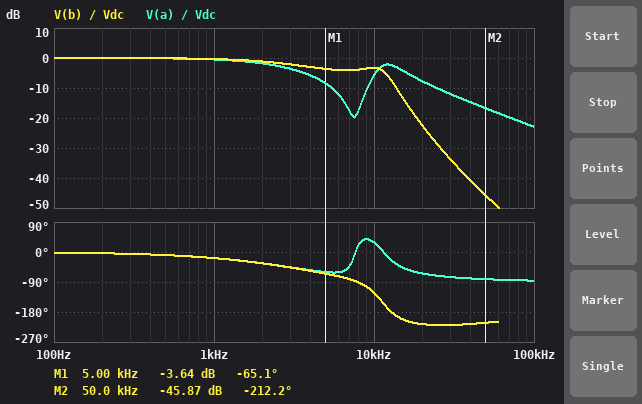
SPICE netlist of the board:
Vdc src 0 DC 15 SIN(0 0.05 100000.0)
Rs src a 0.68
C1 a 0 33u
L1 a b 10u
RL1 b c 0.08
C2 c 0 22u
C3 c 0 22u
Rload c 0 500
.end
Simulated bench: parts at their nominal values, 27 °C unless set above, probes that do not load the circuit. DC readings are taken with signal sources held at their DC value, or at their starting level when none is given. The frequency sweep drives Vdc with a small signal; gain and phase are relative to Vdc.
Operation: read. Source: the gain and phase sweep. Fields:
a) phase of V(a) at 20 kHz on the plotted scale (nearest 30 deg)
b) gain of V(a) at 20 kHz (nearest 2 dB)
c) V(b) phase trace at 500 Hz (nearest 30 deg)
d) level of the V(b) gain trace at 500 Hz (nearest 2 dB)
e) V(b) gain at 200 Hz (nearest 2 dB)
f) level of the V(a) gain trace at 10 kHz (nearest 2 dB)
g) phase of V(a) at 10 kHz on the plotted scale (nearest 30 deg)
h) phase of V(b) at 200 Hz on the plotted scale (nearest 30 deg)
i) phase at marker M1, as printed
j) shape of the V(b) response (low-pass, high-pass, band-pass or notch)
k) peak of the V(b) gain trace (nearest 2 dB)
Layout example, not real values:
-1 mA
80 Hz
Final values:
-60 deg
-8 dB
0 deg
0 dB
0 dB
-6 dB
30 deg
0 deg
-65.1 deg
low-pass
0 dB
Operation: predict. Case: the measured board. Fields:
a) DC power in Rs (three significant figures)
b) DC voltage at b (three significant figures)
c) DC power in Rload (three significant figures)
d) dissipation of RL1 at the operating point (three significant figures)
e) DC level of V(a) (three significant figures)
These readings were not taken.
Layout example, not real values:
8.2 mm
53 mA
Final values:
610 µW
15.0 V
449 mW
71.8 µW
15.0 V
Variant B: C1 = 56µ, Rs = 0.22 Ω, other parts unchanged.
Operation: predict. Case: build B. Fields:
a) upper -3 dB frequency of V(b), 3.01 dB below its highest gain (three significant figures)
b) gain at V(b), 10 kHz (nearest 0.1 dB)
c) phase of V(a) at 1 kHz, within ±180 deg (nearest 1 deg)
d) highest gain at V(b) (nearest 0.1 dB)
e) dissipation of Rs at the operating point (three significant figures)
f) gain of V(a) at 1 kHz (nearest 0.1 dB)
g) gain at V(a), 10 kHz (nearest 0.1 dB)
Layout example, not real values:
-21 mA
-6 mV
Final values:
9.86 kHz
0.7 dB
-8 deg
4.1 dB
198 µW
-0.1 dB
-1.8 dB
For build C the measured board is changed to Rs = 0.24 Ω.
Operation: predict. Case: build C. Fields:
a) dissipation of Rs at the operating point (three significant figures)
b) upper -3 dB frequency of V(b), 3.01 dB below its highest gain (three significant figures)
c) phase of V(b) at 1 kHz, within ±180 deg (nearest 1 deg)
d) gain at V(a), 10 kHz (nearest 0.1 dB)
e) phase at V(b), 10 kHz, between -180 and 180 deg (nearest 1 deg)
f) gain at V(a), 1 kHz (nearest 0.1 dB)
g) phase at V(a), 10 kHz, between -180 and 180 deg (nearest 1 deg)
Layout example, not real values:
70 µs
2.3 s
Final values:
216 µW
9.87 kHz
-7 deg
-2.2 dB
-136 deg
-0.1 dB
15 deg
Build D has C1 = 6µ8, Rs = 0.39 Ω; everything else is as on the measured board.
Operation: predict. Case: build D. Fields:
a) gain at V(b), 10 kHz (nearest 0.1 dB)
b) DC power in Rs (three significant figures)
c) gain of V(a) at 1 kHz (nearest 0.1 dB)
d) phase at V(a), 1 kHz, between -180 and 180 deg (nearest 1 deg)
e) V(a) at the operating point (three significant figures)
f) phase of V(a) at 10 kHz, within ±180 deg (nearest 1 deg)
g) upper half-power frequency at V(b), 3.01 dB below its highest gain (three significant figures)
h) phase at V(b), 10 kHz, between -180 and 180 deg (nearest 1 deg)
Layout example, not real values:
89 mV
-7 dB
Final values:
-2.8 dB
350 µW
-0.1 dB
-7 deg
15.0 V
40 deg
9.42 kHz
-111 deg
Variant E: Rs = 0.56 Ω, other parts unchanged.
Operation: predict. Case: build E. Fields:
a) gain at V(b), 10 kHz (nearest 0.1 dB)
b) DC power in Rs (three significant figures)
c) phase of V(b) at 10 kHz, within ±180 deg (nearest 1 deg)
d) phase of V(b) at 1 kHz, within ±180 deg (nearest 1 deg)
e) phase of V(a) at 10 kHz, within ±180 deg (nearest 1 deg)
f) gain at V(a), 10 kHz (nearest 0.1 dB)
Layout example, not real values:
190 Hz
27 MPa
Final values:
-2.4 dB
503 µW
-125 deg
-15 deg
26 deg
-4.9 dB
